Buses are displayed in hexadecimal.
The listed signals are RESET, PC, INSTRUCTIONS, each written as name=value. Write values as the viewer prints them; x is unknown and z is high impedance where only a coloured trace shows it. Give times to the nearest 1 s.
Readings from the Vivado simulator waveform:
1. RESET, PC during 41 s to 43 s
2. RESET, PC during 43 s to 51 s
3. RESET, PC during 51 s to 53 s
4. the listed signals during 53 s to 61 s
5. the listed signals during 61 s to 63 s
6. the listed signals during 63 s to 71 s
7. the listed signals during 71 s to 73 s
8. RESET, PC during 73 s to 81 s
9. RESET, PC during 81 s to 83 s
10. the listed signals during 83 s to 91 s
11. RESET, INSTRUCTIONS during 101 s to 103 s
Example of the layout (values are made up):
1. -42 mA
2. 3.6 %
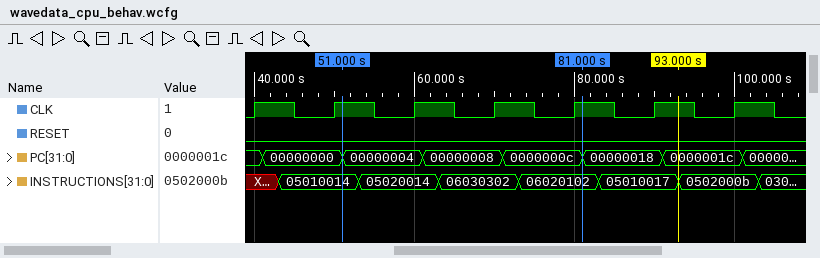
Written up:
1. RESET=0, PC=00000000
2. RESET=0, PC=00000000
3. RESET=0, PC=00000004
4. RESET=0, PC=00000004, INSTRUCTIONS=05020014
5. RESET=0, PC=00000008, INSTRUCTIONS=05020014
6. RESET=0, PC=00000008, INSTRUCTIONS=06030302
7. RESET=0, PC=0000000c, INSTRUCTIONS=06030302
8. RESET=0, PC=0000000c
9. RESET=0, PC=00000018
10. RESET=0, PC=00000018, INSTRUCTIONS=05010017
11. RESET=0, INSTRUCTIONS=0502000b
